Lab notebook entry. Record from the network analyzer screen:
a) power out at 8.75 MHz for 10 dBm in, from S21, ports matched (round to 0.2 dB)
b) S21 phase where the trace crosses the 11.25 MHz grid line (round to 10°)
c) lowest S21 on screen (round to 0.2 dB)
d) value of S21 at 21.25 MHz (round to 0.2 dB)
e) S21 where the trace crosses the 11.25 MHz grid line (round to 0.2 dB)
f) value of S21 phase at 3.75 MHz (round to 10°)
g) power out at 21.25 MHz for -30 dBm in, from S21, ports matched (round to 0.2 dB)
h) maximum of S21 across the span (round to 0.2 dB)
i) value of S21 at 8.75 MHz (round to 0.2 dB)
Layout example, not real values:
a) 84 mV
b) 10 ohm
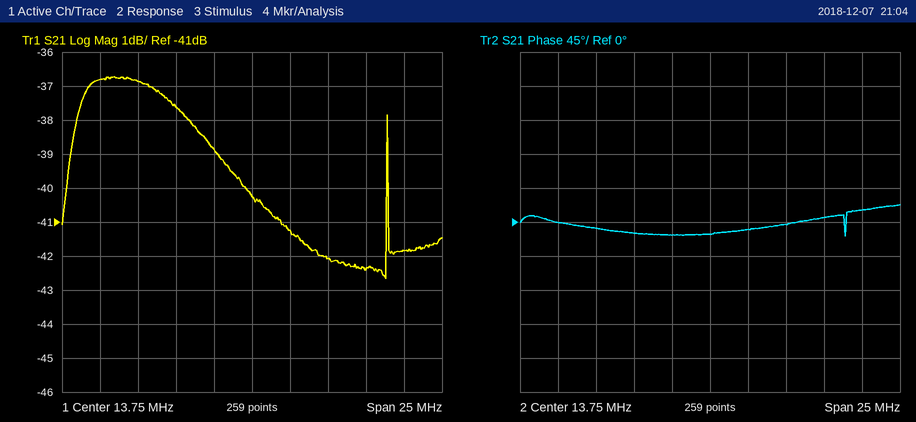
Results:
a) -27.6 dBm
b) -20°
c) -42.6 dB
d) -42.4 dB
e) -38.8 dB
f) 0°
g) -72.4 dBm
h) -36.8 dB
i) -37.6 dB
